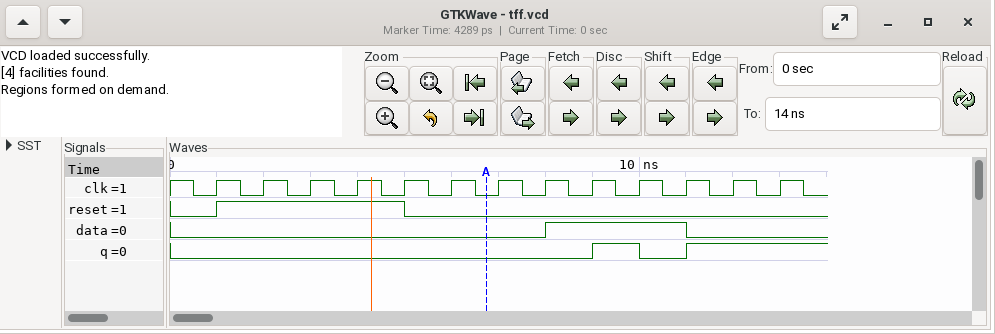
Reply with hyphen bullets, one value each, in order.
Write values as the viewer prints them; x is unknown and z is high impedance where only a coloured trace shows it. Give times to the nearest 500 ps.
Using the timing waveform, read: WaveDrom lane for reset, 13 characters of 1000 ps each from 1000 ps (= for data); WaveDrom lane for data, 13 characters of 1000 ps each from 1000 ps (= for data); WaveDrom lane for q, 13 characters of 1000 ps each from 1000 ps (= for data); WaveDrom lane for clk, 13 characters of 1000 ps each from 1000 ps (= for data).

- {name: 'reset', wave: '1...0........'}
- {name: 'data', wave: '0......1..0..'}
- {name: 'q', wave: '0.......101..'}
- {name: 'clk', wave: 'p............'}
